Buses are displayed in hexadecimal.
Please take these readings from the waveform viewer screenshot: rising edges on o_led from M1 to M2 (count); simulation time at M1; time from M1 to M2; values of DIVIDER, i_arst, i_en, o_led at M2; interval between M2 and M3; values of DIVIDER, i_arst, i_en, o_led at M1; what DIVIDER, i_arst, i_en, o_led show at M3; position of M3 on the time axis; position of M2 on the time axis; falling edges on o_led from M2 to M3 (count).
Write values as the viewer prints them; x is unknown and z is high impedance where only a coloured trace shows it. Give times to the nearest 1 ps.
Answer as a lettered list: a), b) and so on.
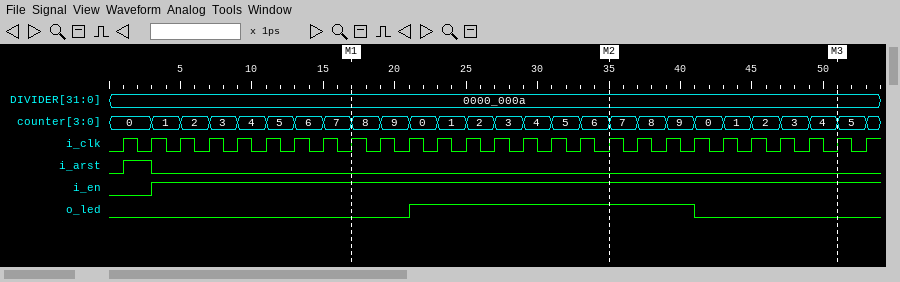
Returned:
a) 1
b) 17 ps
c) 18 ps
d) DIVIDER=0000_000a, i_arst=0, i_en=1, o_led=1
e) 16 ps
f) DIVIDER=0000_000a, i_arst=0, i_en=1, o_led=0
g) DIVIDER=0000_000a, i_arst=0, i_en=1, o_led=0
h) 51 ps
i) 35 ps
j) 1
